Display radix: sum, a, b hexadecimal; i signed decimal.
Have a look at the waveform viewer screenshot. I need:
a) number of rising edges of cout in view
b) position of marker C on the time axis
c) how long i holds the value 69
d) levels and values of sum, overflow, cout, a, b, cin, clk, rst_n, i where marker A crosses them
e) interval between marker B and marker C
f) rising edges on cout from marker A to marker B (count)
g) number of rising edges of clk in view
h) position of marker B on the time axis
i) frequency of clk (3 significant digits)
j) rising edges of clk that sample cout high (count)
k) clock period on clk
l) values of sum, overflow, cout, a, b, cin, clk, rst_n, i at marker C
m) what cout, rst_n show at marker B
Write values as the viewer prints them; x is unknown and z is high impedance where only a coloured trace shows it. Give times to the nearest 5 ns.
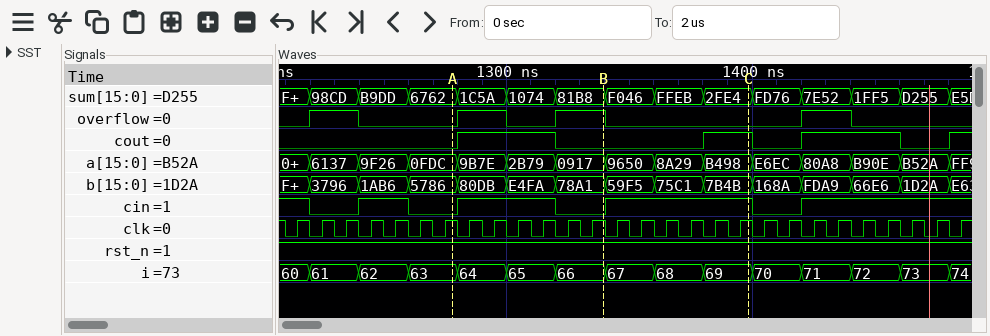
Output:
4
1400 ns
20 ns
sum=6762, overflow=0, cout=0, a=0FDC, b=5786, cin=0, clk=1, rst_n=1, i=63
60 ns
1
28
1340 ns
100 MHz
11
10 ns
sum=2FE4, overflow=0, cout=1, a=B498, b=7B4B, cin=1, clk=1, rst_n=1, i=69
cout=0, rst_n=1
